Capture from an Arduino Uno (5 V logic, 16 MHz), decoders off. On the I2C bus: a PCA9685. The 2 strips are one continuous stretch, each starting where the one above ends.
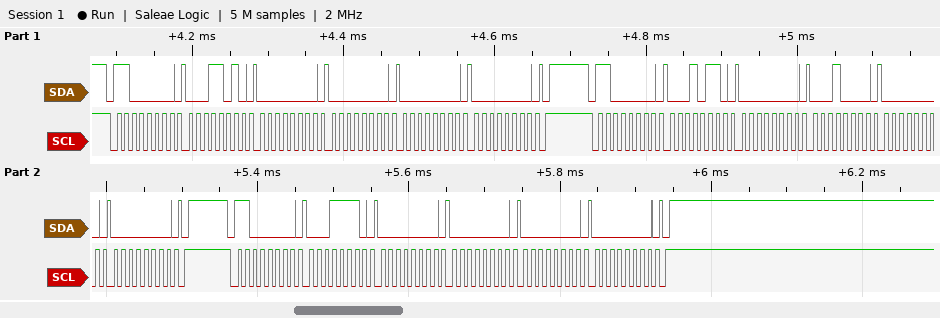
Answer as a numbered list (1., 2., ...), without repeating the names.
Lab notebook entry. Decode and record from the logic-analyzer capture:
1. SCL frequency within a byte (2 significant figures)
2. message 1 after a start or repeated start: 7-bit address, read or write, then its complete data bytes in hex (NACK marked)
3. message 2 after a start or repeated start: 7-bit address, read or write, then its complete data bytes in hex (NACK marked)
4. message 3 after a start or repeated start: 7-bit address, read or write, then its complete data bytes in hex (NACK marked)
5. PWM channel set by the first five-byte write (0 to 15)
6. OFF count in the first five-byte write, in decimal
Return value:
1. 100 kHz
2. 0x60 write: 1A 00 00 00 00
3. 0x60 write: 16 00 10 00 00
4. 0x60 write: 1E 00 00 00 00
5. 5
6. 0
